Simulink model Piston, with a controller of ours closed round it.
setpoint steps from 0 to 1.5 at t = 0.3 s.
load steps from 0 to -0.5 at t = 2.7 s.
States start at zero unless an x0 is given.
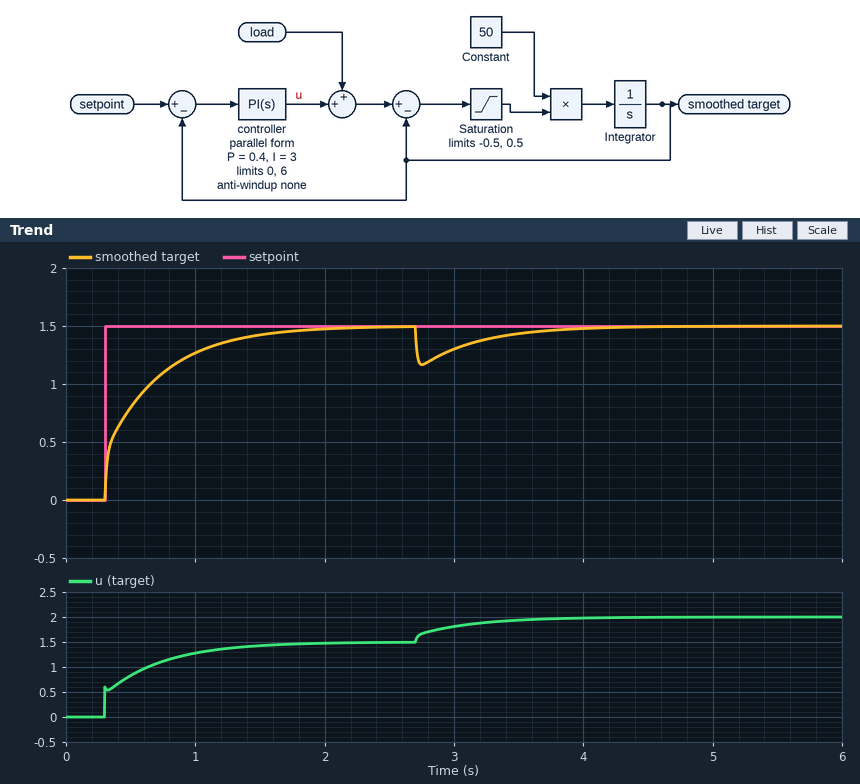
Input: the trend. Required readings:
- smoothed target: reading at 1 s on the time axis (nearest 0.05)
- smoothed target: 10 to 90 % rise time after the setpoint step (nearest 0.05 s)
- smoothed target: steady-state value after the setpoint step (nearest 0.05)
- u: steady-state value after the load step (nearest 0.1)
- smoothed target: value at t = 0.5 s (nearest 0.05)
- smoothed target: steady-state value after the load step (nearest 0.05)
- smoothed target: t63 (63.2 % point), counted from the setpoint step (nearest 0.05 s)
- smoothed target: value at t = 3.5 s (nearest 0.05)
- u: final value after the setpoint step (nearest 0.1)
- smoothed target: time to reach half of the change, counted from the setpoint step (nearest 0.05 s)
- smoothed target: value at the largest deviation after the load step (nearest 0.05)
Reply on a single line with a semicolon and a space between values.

1.25; 0.90 s; 1.50; 2.0; 0.80; 1.50; 0.30 s; 1.45; 1.5; 0.15 s; 1.15
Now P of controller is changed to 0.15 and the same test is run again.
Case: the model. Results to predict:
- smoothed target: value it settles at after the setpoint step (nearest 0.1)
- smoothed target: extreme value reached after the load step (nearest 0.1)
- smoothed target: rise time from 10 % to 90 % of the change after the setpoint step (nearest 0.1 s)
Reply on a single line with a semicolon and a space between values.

1.5; 1.1; 0.8 s
